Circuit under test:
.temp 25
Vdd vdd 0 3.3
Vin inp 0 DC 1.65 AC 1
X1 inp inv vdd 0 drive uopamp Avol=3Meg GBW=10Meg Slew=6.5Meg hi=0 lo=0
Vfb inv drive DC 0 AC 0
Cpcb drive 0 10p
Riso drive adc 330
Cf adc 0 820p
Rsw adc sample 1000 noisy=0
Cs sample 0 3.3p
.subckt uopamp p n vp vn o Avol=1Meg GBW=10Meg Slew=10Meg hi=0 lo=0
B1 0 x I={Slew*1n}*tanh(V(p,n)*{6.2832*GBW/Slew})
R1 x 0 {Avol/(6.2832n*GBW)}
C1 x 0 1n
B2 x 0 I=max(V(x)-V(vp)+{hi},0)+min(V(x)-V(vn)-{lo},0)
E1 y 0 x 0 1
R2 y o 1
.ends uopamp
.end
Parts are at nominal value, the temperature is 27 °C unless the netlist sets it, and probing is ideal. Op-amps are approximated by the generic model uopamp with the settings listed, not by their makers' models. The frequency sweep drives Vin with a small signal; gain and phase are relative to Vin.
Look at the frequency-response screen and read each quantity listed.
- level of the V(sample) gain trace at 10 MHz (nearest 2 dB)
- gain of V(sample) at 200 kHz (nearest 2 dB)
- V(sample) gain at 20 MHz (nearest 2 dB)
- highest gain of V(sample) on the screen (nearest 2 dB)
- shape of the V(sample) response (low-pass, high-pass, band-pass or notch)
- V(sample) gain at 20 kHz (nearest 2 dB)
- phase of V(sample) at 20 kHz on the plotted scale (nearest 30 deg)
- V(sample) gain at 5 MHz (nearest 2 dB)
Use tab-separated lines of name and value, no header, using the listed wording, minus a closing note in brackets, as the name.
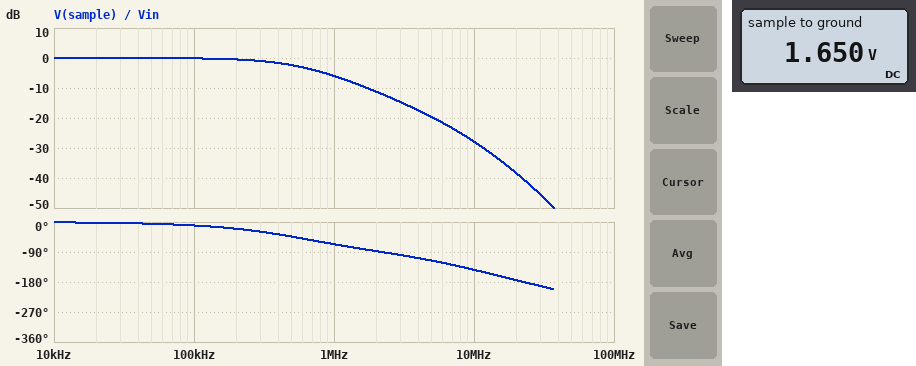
level of the V(sample) gain trace at 10 MHz	-28 dB
gain of V(sample) at 200 kHz	0 dB
V(sample) gain at 20 MHz	-38 dB
highest gain of V(sample) on the screen	0 dB
shape of the V(sample) response	low-pass
V(sample) gain at 20 kHz	0 dB
phase of V(sample) at 20 kHz on the plotted scale	0 deg
V(sample) gain at 5 MHz	-20 dB
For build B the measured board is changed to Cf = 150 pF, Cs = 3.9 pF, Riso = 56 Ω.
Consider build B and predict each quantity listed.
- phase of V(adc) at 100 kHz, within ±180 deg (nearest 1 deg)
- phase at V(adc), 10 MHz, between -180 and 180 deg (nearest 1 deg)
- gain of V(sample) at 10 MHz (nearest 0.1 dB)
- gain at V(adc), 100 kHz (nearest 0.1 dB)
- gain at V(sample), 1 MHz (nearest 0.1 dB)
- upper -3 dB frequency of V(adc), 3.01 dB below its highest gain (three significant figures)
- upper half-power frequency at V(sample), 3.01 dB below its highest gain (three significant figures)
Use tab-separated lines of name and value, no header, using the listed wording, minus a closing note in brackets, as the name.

phase of V(adc) at 100 kHz, within ±180 deg	-1 deg
phase at V(adc), 10 MHz, between -180 and 180 deg	-74 deg
gain of V(sample) at 10 MHz	-4.4 dB
gain at V(adc), 100 kHz	0 dB
gain at V(sample), 1 MHz	-0.1 dB
upper -3 dB frequency of V(adc), 3.01 dB below its highest gain	8.20 MHz
upper half-power frequency at V(sample), 3.01 dB below its highest gain	7.93 MHz
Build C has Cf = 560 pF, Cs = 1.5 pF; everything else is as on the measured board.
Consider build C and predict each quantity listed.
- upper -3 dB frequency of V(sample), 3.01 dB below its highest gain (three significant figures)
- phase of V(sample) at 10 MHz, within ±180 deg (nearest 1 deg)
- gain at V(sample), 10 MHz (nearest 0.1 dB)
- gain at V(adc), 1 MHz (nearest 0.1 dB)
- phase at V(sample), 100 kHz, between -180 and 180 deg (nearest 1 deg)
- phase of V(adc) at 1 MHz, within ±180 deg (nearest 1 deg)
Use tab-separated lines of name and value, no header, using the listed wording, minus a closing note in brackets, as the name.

upper -3 dB frequency of V(sample), 3.01 dB below its highest gain	853 kHz
phase of V(sample) at 10 MHz, within ±180 deg	-136 deg
gain at V(sample), 10 MHz	-24.4 dB
gain at V(adc), 1 MHz	-3.8 dB
phase at V(sample), 100 kHz, between -180 and 180 deg	-7 deg
phase of V(adc) at 1 MHz, within ±180 deg	-55 deg
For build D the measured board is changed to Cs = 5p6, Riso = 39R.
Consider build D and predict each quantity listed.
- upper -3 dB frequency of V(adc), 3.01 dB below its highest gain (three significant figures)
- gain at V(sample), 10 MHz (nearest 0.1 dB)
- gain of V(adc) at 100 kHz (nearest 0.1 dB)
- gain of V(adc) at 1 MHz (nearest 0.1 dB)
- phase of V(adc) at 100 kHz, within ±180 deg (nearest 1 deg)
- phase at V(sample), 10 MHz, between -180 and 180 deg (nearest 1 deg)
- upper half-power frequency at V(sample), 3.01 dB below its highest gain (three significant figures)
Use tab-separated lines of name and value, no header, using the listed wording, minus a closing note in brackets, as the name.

upper -3 dB frequency of V(adc), 3.01 dB below its highest gain	4.17 MHz
gain at V(sample), 10 MHz	-10.6 dB
gain of V(adc) at 100 kHz	0 dB
gain of V(adc) at 1 MHz	-0.2 dB
phase of V(adc) at 100 kHz, within ±180 deg	-2 deg
phase at V(sample), 10 MHz, between -180 and 180 deg	-129 deg
upper half-power frequency at V(sample), 3.01 dB below its highest gain	4.10 MHz
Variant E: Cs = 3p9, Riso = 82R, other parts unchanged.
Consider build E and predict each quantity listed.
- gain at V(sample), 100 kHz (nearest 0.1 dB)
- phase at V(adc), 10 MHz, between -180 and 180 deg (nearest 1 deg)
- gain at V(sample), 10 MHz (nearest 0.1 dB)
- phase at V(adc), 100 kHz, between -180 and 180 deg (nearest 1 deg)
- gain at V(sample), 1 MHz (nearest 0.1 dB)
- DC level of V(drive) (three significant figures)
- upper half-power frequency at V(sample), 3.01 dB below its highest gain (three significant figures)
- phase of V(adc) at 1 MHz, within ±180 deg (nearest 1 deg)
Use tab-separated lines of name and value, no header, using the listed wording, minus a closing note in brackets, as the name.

gain at V(sample), 100 kHz	0 dB
phase at V(adc), 10 MHz, between -180 and 180 deg	-122 deg
gain at V(sample), 10 MHz	-16.1 dB
phase at V(adc), 100 kHz, between -180 and 180 deg	-3 deg
gain at V(sample), 1 MHz	-0.8 dB
DC level of V(drive)	1.65 V
upper half-power frequency at V(sample), 3.01 dB below its highest gain	2.24 MHz
phase of V(adc) at 1 MHz, within ±180 deg	-29 deg
